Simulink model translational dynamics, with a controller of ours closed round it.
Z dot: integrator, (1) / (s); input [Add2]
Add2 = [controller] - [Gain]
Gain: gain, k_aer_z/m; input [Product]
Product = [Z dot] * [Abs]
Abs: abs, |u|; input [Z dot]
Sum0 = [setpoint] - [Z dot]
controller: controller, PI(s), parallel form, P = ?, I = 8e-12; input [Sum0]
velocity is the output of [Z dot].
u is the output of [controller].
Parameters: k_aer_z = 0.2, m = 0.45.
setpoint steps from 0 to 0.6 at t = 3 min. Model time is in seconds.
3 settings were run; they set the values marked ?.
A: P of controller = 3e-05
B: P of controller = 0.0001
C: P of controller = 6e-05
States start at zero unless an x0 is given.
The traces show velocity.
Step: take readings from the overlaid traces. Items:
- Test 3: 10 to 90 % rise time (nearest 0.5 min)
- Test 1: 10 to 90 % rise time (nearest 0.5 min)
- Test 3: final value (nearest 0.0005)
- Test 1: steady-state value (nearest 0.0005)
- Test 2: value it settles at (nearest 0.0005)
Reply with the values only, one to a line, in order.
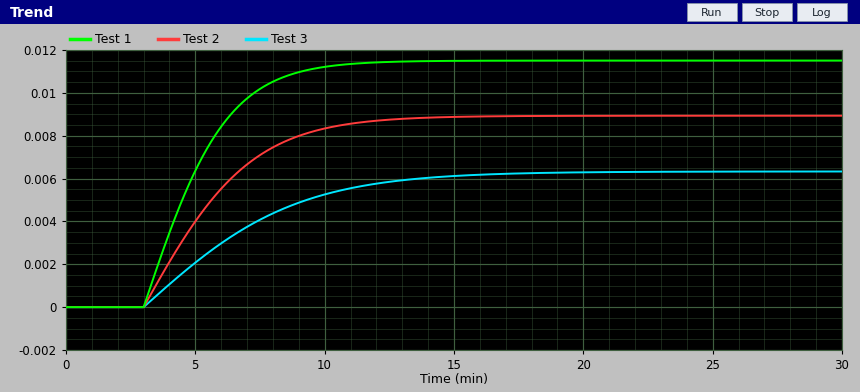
8.0 min
4.5 min
0.0065
0.0115
0.0090
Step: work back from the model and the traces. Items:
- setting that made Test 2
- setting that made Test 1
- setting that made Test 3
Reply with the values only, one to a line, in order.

C
B
A
